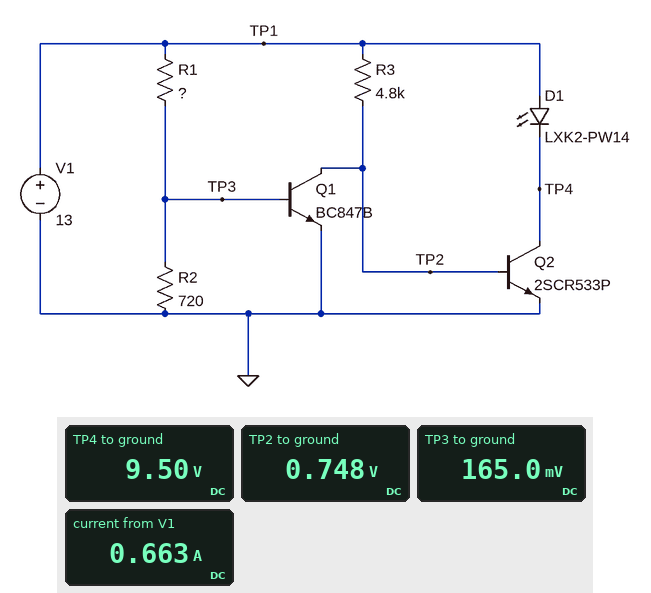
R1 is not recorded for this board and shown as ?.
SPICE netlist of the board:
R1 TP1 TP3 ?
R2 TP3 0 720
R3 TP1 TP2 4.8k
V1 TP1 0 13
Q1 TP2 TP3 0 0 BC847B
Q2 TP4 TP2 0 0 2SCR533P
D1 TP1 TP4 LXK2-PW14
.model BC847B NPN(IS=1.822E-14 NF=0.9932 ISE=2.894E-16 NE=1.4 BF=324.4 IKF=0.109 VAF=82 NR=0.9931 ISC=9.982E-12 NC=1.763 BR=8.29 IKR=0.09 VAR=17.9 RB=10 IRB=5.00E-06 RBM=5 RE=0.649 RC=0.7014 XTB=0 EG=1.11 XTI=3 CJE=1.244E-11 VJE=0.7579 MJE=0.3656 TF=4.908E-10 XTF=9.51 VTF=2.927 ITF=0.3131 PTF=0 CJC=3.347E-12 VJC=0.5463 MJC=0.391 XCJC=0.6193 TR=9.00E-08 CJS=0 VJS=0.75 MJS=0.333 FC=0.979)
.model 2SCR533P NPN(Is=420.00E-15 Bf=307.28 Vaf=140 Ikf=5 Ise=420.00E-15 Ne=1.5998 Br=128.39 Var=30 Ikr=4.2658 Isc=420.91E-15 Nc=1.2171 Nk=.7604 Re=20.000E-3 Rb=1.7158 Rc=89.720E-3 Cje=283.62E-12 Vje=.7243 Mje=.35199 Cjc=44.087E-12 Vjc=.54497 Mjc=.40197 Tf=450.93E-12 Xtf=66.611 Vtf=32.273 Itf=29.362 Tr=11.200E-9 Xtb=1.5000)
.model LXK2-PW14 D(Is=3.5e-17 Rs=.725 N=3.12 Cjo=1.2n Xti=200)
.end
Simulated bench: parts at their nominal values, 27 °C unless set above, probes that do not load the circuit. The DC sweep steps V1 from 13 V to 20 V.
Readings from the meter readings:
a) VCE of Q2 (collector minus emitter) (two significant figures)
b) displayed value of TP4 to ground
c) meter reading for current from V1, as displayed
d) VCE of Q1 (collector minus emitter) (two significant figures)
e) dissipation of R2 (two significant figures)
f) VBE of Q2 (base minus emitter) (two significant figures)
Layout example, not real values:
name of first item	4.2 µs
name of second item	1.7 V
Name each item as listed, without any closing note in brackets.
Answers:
VCE of Q2 (collector minus emitter)	9.5 V
displayed value of TP4 to ground	9.50 V
meter reading for current from V1, as displayed	0.663 A
VCE of Q1 (collector minus emitter)	750 mV
dissipation of R2	38 µW
VBE of Q2 (base minus emitter)	750 mV
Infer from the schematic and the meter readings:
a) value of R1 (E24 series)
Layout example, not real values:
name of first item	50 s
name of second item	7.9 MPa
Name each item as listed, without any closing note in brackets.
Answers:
value of R1	56 kΩ
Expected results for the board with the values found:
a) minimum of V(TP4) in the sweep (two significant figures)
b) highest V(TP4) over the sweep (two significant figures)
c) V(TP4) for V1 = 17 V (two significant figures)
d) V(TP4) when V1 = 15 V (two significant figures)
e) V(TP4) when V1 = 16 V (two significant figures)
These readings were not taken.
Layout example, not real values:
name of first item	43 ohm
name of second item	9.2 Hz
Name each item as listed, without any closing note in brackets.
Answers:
minimum of V(TP4) in the sweep	9.5 V
highest V(TP4) over the sweep	16 V
V(TP4) for V1 = 17 V	13 V
V(TP4) when V1 = 15 V	11 V
V(TP4) when V1 = 16 V	12 V
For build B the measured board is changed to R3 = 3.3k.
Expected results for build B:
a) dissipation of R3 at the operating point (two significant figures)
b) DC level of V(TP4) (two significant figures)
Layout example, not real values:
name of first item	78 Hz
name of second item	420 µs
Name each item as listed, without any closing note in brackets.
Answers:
dissipation of R3 at the operating point	45 mW
DC level of V(TP4)	9.3 V
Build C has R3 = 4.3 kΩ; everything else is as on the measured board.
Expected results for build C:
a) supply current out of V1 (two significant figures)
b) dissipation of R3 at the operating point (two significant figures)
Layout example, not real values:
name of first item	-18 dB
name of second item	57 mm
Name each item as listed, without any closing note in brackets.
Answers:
supply current out of V1	730 mA
dissipation of R3 at the operating point	35 mW
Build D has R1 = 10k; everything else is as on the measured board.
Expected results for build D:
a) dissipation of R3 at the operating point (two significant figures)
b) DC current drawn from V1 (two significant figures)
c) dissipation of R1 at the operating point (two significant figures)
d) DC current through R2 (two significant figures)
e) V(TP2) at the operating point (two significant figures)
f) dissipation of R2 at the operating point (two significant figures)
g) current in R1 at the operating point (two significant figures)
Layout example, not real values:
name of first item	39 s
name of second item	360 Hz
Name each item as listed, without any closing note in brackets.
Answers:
dissipation of R3 at the operating point	35 mW
DC current drawn from V1	3.9 mA
dissipation of R1 at the operating point	15 mW
DC current through R2	950 µA
V(TP2) at the operating point	28 mV
dissipation of R2 at the operating point	650 µW
current in R1 at the operating point	1.2 mA
